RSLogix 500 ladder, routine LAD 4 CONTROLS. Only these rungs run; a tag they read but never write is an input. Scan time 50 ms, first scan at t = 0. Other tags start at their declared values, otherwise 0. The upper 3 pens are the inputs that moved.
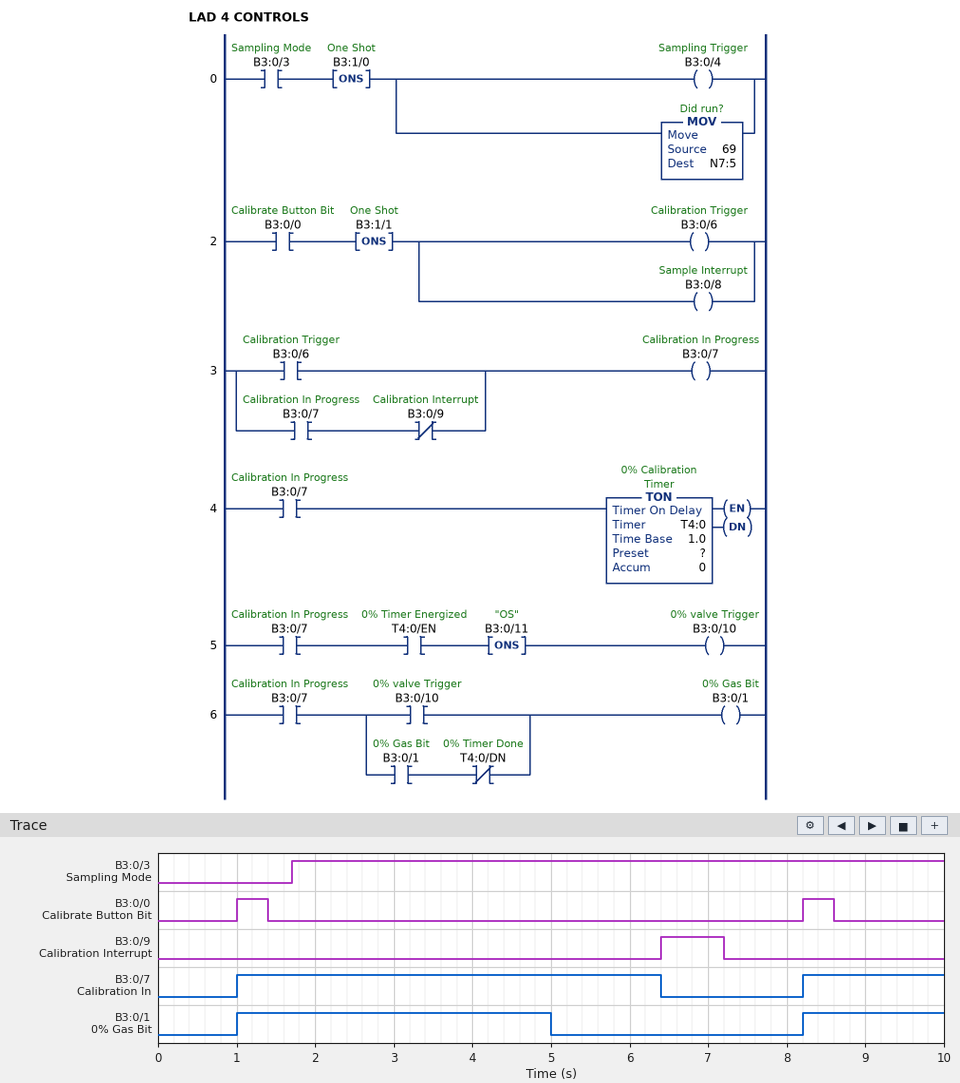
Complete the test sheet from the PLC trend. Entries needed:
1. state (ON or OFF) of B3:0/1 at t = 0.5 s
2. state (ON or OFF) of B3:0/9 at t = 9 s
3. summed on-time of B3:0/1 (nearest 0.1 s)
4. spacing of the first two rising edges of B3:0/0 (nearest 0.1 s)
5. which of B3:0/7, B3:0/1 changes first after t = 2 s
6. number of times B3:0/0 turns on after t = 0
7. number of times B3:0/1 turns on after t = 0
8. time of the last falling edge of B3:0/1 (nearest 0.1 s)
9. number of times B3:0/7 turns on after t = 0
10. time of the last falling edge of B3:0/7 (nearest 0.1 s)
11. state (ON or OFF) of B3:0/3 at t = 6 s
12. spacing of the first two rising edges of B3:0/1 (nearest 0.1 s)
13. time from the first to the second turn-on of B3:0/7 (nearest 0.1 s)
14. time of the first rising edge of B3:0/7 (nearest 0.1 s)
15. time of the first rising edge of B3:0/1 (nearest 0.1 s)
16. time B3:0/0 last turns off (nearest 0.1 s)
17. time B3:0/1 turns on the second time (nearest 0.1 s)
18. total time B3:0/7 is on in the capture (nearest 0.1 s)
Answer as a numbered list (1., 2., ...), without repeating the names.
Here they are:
1. OFF
2. OFF
3. 5.8 s
4. 7.2 s
5. B3:0/1
6. 2
7. 2
8. 5.0 s
9. 2
10. 6.4 s
11. ON
12. 7.2 s
13. 7.2 s
14. 1.0 s
15. 1.0 s
16. 8.6 s
17. 8.2 s
18. 7.2 s
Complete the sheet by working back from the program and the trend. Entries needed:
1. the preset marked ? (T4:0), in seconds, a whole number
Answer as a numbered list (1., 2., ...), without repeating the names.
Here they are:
1. 4 s
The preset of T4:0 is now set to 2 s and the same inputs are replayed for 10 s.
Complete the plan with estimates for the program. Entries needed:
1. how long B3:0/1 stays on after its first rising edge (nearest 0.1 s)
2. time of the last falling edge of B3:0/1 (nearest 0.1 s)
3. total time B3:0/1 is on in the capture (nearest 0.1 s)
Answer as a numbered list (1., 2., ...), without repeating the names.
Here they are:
1. 2.0 s
2. 3.0 s
3. 3.8 s
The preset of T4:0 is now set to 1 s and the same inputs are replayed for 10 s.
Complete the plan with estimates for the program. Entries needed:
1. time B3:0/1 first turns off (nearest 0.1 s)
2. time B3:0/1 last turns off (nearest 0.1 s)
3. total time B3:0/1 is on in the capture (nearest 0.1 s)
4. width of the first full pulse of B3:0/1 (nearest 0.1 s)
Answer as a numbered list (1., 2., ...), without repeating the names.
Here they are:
1. 2.0 s
2. 9.2 s
3. 2.0 s
4. 1.0 s
